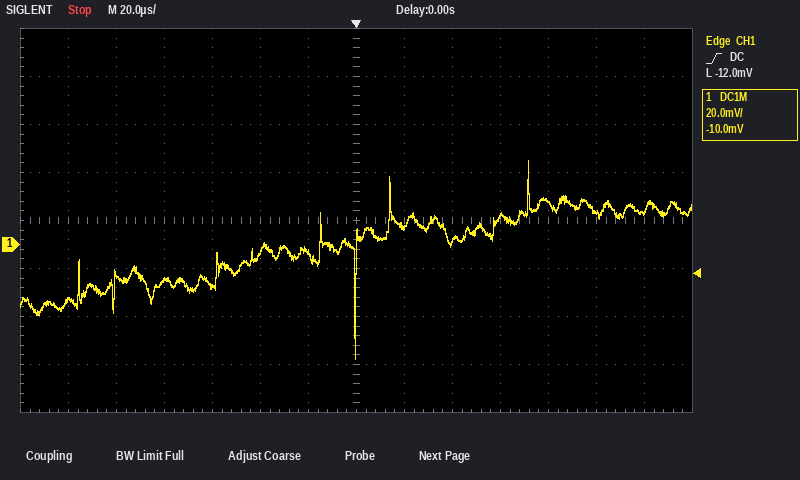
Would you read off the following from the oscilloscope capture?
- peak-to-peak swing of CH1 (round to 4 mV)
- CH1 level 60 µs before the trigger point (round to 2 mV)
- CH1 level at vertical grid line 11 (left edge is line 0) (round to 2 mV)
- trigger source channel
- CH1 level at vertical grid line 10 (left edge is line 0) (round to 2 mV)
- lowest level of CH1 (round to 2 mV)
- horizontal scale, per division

84 mV
-18 mV
18 mV
CH1
12 mV
-48 mV
20 µs
